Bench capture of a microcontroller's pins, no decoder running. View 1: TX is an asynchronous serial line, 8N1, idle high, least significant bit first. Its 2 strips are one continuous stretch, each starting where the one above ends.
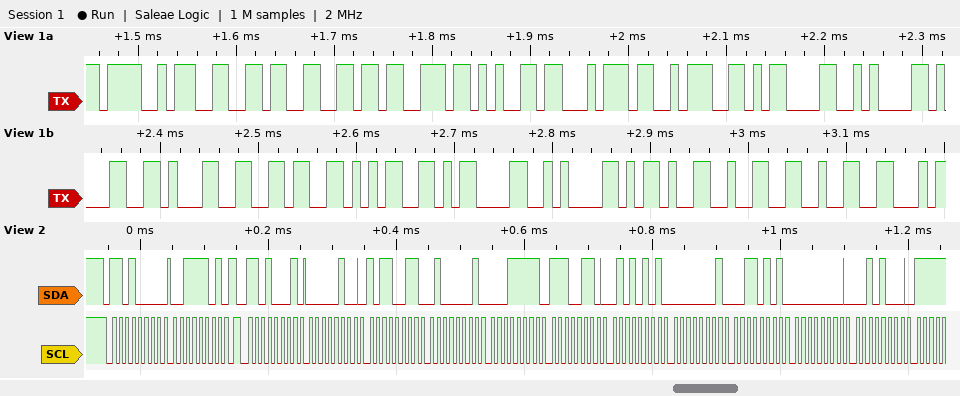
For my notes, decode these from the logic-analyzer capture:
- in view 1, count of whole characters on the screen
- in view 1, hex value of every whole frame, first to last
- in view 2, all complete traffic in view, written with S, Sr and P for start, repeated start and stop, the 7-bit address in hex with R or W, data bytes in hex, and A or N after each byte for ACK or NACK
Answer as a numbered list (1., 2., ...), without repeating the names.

1. 18
2. 0x4F 0x66 0x66 0x73 0x65 0x74 0x3A 0x0D 0x0A 0x31 0x31 0x36 0x35 0x0D 0x0A 0x2D 0x32 0x32
3. S 68W A 3D A Sr 68R A 04 A B3 A 41 A 1F A E6 A 55 A 01 A 35 A 00 A 28 A
